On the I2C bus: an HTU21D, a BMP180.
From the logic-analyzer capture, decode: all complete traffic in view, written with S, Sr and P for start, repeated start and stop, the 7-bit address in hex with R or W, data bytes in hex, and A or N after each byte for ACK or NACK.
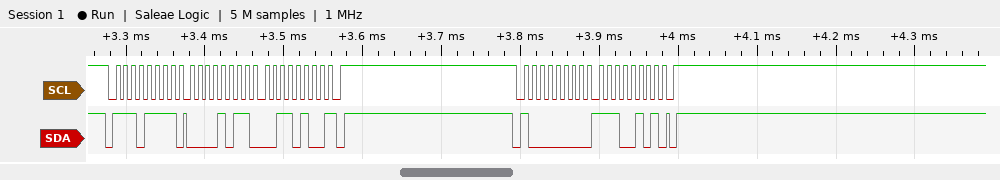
S 77R A 0B A 34 N P S 40W A E5 A P
